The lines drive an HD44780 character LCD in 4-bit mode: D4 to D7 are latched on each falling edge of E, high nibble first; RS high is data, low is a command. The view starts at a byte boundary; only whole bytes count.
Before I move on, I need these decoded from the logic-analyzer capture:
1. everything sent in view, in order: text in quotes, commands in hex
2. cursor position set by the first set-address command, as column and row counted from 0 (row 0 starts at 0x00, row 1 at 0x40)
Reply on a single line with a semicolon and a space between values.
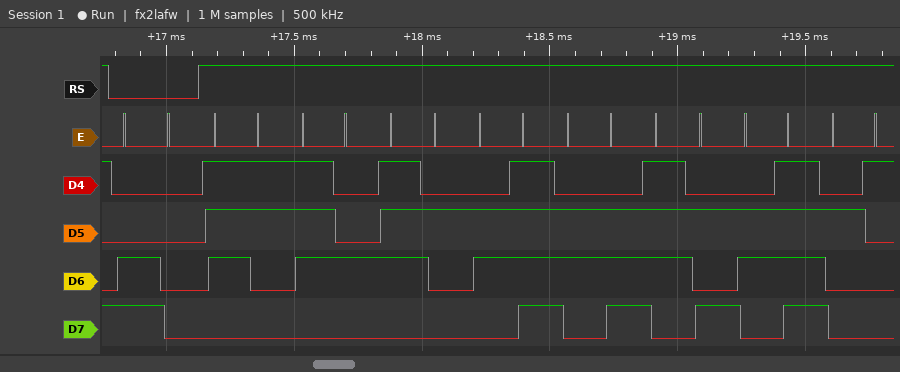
0xC0 "stronzo!"; column 0, row 1
